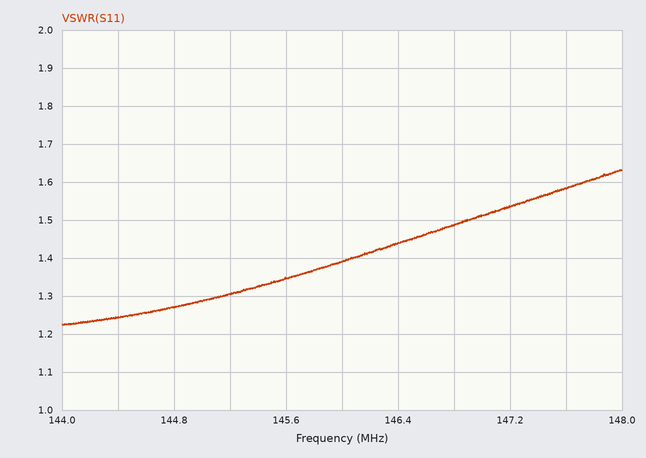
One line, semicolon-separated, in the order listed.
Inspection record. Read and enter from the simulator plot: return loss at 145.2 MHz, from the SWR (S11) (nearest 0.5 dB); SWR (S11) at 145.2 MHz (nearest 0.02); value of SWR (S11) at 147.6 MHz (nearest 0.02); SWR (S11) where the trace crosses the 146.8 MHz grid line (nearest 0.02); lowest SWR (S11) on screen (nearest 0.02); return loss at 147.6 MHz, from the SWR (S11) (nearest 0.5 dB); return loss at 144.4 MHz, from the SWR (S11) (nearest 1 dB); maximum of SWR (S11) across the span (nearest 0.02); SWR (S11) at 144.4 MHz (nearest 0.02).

17.5 dB; 1.30; 1.58; 1.48; 1.22; 13.0 dB; 19 dB; 1.64; 1.24
